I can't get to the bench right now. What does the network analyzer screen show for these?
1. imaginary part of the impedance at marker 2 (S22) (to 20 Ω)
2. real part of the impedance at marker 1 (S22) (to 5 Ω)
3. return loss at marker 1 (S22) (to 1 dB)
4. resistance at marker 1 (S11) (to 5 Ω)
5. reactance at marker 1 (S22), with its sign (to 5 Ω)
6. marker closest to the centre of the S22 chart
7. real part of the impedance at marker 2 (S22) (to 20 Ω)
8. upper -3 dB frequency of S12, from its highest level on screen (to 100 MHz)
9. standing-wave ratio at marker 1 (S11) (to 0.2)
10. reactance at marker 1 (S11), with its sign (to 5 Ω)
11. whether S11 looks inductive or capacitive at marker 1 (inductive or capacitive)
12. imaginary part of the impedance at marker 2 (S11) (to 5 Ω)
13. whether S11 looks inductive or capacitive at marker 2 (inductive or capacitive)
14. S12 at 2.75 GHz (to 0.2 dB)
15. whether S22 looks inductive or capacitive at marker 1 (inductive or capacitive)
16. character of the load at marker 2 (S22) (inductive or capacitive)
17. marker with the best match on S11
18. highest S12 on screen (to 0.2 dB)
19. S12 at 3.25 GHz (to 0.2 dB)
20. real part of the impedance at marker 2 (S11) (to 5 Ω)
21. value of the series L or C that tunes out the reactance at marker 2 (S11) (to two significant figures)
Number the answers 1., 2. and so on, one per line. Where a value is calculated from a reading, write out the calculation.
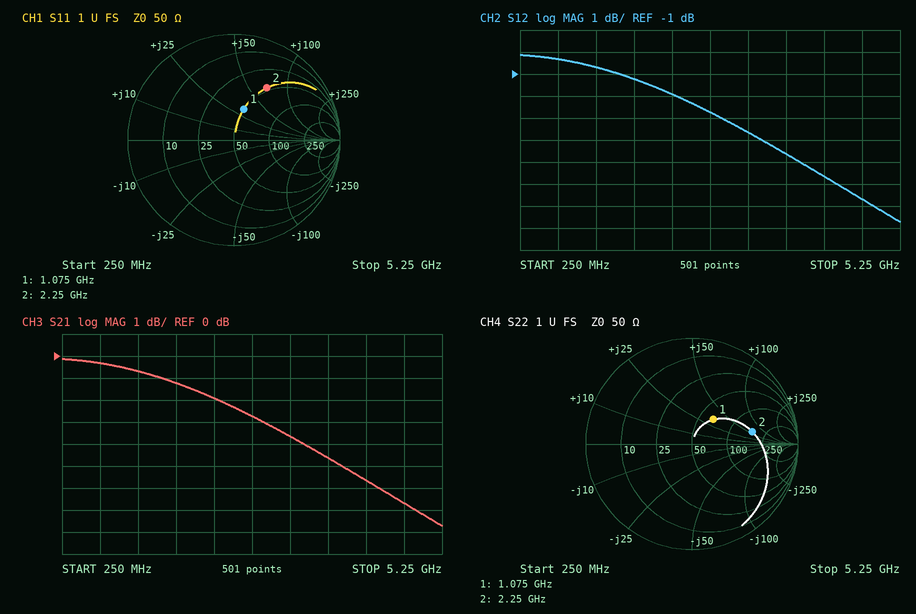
1. +60 Ω
2. 65 Ω
3. 10 dB
4. 50 Ω
5. +35 Ω
6. marker 1
7. 160 Ω
8. 3.0 GHz
9. 1.8
10. +30 Ω
11. inductive
12. +70 Ω
13. inductive
14. -2.8 dB
15. inductive
16. inductive
17. marker 1
18. -0.2 dB
19. -3.6 dB
20. 45 Ω
21. C = 1/(2π × 2.25 GHz × 70 Ω) ≈ 1.0 pF
